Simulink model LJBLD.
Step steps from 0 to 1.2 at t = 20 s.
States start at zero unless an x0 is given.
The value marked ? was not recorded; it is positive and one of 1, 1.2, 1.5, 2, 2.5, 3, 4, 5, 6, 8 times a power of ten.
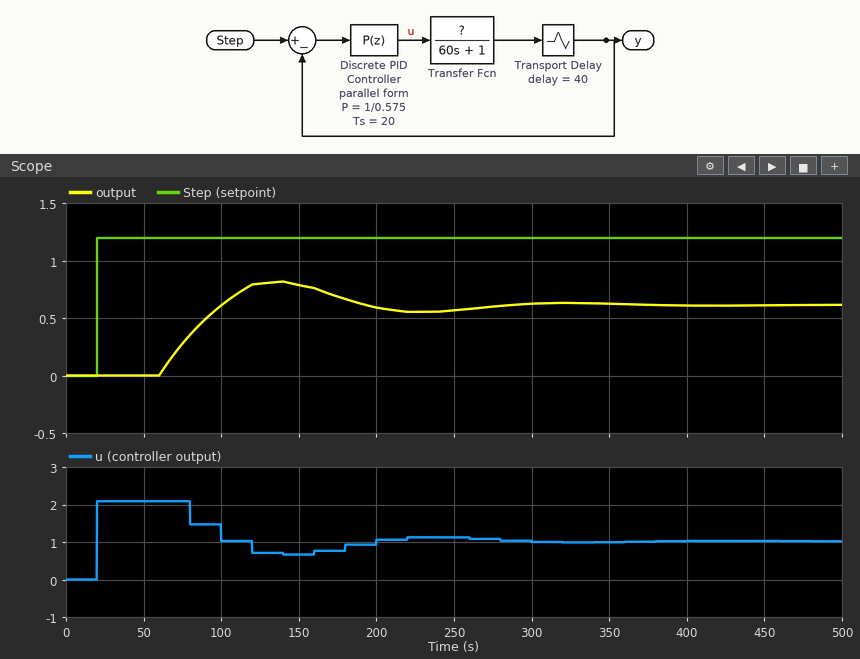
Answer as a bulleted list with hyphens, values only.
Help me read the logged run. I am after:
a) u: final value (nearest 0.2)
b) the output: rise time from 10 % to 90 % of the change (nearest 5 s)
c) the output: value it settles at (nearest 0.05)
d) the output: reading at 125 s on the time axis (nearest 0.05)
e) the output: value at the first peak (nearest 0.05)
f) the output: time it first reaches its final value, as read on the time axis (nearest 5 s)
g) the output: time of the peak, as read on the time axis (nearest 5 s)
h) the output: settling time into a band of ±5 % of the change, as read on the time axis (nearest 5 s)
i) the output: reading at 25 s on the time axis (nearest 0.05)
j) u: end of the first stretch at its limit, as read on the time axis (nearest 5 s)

- 1.0
- 30 s
- 0.60
- 0.80
- 0.80
- 100 s
- 140 s
- 265 s
- 0.00
- 80 s
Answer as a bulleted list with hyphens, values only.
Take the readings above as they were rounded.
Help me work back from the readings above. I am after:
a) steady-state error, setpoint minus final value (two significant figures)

- 0.60
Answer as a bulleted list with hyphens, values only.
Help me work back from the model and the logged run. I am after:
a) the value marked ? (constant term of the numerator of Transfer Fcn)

- 0.6
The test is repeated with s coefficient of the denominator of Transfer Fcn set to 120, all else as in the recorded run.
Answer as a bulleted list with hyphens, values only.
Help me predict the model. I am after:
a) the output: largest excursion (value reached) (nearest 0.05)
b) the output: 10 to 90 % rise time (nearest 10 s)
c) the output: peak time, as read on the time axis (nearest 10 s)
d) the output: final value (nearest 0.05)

- 0.65
- 70 s
- 200 s
- 0.60
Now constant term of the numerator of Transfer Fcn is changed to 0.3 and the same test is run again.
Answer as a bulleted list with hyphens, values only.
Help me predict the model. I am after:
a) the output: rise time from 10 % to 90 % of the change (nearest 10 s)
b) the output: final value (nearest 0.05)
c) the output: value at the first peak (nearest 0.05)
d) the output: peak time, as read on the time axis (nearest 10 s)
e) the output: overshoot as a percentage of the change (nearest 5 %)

- 50 s
- 0.40
- 0.45
- 160 s
- 10 %
